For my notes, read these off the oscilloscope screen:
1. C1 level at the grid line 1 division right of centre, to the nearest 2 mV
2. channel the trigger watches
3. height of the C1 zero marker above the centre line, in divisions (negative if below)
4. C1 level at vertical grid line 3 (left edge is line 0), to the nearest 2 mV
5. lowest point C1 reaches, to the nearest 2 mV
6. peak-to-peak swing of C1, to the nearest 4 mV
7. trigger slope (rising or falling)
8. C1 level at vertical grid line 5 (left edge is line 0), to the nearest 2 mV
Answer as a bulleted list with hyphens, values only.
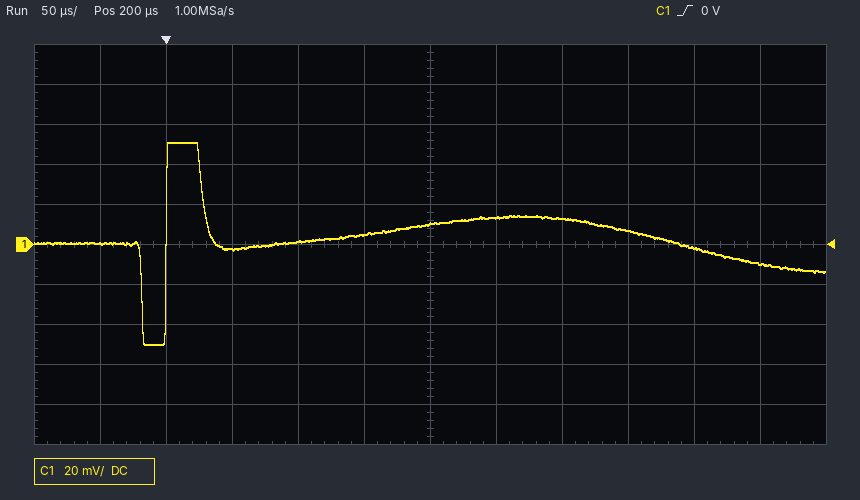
- 14 mV
- C1
- 0.0 div
- -2 mV
- -50 mV
- 100 mV
- rising
- 4 mV
